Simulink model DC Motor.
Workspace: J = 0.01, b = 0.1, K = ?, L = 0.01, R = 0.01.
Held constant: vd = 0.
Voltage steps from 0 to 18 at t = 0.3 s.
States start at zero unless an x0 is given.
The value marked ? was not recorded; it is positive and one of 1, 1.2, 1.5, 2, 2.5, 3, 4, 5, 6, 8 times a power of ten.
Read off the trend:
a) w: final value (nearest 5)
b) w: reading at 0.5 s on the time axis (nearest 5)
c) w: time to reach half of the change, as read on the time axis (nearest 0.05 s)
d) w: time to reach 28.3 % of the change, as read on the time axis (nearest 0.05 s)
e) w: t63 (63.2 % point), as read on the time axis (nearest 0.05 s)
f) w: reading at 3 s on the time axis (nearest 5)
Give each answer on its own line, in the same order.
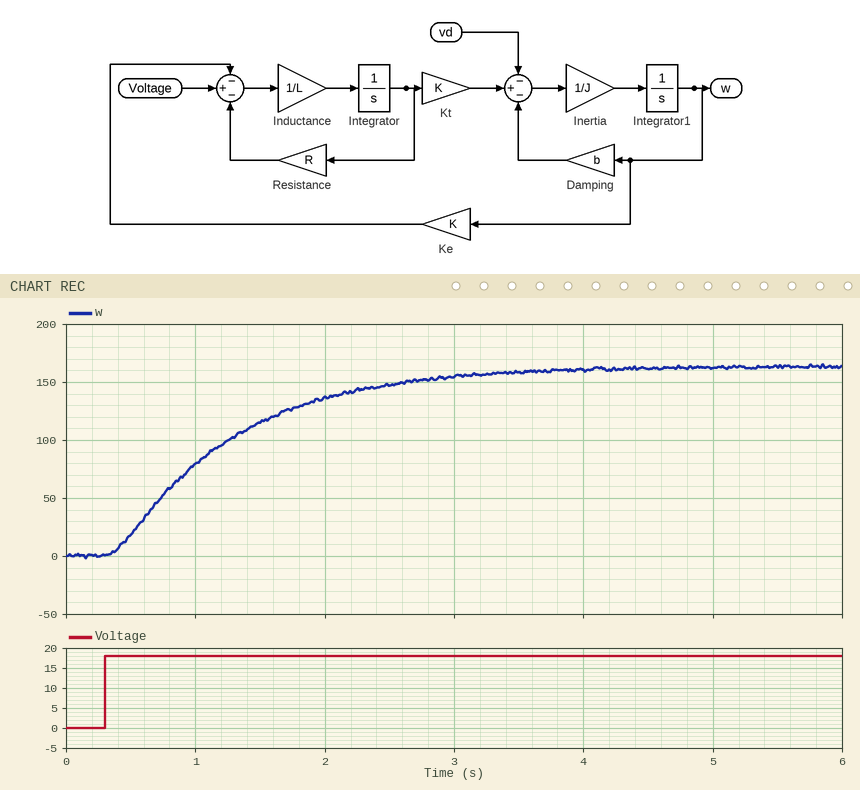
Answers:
165
20
1.05 s
0.70 s
1.30 s
155
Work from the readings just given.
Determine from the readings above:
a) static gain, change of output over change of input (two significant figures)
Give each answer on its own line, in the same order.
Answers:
9.2
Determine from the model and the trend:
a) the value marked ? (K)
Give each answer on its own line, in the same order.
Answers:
0.01
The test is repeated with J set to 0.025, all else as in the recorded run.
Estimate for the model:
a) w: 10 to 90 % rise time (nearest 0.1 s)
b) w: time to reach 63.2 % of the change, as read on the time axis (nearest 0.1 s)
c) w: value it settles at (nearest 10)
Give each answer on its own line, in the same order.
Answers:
2.1 s
1.5 s
160
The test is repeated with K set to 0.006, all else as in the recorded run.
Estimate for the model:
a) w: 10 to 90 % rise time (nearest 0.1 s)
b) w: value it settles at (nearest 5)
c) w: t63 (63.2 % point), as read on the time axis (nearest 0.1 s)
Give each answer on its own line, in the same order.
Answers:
2.1 s
105
1.4 s
